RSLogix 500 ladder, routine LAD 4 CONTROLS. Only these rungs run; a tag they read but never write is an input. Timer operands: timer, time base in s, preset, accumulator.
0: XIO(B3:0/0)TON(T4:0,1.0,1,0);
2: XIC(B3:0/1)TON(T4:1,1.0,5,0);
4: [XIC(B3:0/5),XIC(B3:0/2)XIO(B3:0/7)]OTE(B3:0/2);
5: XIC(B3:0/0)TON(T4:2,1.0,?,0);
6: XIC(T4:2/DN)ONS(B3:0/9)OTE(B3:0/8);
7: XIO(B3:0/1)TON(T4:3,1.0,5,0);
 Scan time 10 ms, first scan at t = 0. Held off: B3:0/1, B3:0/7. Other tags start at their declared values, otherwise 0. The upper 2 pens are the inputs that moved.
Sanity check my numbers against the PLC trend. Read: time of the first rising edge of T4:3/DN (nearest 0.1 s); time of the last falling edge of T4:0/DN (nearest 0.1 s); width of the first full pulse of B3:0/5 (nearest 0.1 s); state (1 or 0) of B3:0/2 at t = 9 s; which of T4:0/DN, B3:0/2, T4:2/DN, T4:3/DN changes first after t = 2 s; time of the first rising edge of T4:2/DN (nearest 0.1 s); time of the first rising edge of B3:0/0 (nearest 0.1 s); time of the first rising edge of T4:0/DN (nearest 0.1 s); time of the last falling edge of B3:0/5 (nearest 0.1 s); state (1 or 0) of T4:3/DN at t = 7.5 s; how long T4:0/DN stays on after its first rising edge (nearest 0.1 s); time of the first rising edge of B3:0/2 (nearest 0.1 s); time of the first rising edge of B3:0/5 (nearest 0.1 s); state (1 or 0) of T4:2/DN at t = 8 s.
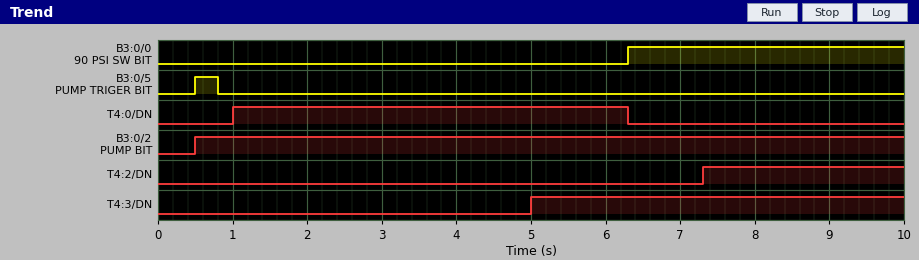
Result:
5.0 s
6.3 s
0.3 s
1
T4:3/DN
7.3 s
6.3 s
1.0 s
0.8 s
1
5.3 s
0.5 s
0.5 s
1
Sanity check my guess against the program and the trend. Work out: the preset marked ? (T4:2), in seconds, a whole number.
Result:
1 s
